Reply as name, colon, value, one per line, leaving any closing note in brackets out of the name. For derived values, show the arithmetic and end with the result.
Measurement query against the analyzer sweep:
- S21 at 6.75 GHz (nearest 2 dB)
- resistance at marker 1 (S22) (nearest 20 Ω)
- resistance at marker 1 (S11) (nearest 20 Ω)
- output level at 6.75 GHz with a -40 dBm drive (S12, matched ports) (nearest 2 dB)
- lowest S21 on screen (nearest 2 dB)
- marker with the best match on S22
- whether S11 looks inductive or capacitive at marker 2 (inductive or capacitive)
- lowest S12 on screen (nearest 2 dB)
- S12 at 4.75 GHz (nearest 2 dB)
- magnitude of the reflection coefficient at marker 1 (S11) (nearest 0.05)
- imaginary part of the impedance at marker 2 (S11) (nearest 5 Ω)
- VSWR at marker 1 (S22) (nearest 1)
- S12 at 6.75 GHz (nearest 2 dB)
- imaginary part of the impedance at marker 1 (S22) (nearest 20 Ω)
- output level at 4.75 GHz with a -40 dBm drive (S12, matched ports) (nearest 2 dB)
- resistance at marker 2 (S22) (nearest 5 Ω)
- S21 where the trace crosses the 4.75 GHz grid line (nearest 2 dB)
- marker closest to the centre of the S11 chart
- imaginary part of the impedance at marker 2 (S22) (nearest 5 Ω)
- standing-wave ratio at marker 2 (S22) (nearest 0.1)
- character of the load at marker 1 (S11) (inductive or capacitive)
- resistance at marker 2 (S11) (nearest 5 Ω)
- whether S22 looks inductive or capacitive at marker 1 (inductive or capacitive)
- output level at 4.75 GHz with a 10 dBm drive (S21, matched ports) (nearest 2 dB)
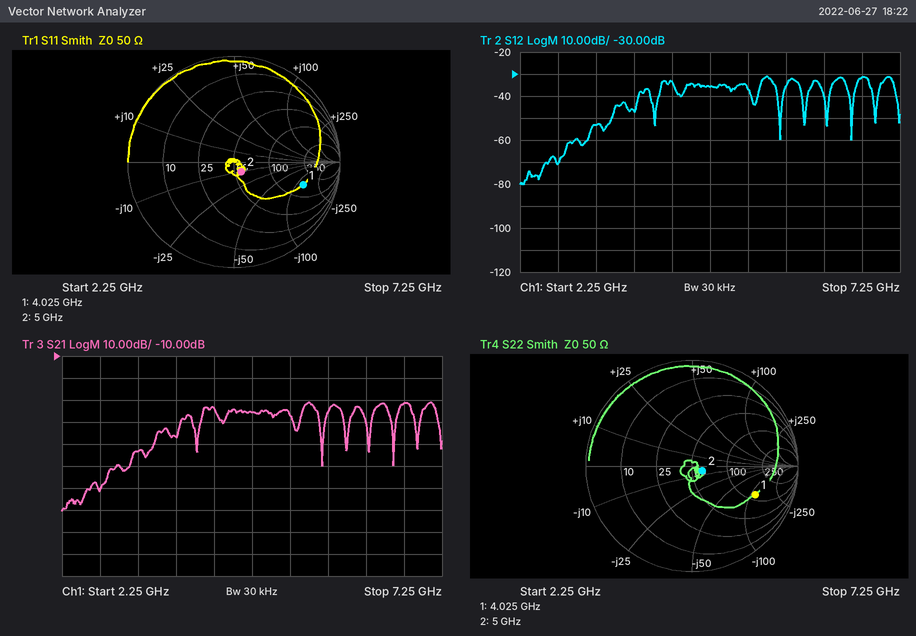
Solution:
S21 at 6.75 GHz: -32 dB
resistance at marker 1 (S22): 120 Ω
resistance at marker 1 (S11): 160 Ω
output level at 6.75 GHz with a -40 dBm drive (S12, matched ports): -40 dBm + (-32 dB) = -72 dBm
lowest S21 on screen: -80 dB
marker with the best match on S22: marker 2
whether S11 looks inductive or capacitive at marker 2: capacitive
lowest S12 on screen: -80 dB
S12 at 4.75 GHz: -36 dB
magnitude of the reflection coefficient at marker 1 (S11): 0.70
imaginary part of the impedance at marker 2 (S11): -10 Ω
VSWR at marker 1 (S22): 5
S12 at 6.75 GHz: -32 dB
imaginary part of the impedance at marker 1 (S22): -120 Ω
output level at 4.75 GHz with a -40 dBm drive (S12, matched ports): -40 dBm + (-36 dB) = -76 dBm
resistance at marker 2 (S22): 60 Ω
S21 where the trace crosses the 4.75 GHz grid line: -36 dB
marker closest to the centre of the S11 chart: marker 2
imaginary part of the impedance at marker 2 (S22): -5 Ω
standing-wave ratio at marker 2 (S22): 1.2
character of the load at marker 1 (S11): capacitive
resistance at marker 2 (S11): 55 Ω
whether S22 looks inductive or capacitive at marker 1: capacitive
output level at 4.75 GHz with a 10 dBm drive (S21, matched ports): 10 dBm + (-36 dB) = -26 dBm
